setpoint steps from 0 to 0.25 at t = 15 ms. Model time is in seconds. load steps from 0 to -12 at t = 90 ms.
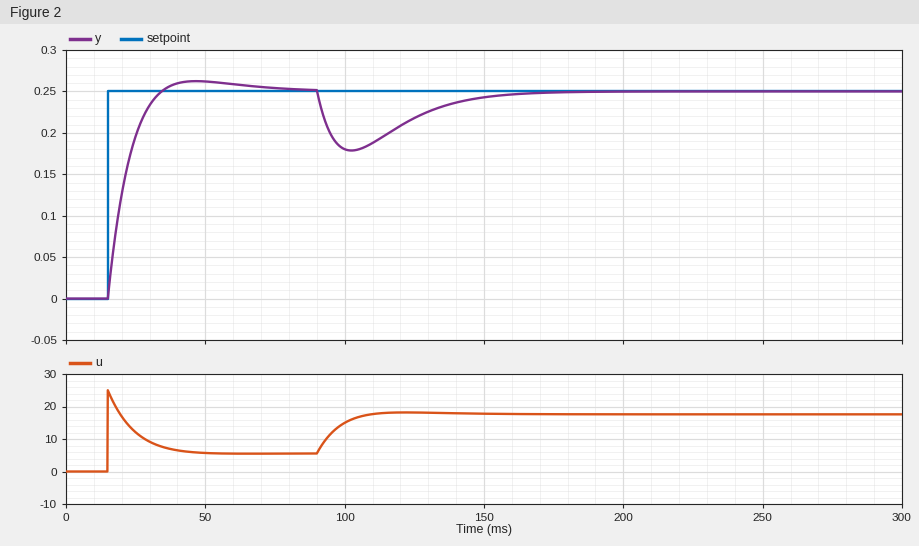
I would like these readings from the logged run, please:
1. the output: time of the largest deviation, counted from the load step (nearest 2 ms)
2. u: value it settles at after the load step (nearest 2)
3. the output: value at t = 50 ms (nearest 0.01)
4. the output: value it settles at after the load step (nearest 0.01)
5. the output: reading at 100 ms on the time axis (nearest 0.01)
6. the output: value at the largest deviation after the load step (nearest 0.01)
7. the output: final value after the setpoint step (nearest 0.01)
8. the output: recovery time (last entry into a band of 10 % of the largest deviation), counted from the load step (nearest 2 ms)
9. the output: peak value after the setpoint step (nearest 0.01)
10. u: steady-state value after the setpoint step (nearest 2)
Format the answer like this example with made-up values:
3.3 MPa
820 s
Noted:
12 ms
18
0.26
0.25
0.18
0.18
0.25
60 ms
0.26
6
